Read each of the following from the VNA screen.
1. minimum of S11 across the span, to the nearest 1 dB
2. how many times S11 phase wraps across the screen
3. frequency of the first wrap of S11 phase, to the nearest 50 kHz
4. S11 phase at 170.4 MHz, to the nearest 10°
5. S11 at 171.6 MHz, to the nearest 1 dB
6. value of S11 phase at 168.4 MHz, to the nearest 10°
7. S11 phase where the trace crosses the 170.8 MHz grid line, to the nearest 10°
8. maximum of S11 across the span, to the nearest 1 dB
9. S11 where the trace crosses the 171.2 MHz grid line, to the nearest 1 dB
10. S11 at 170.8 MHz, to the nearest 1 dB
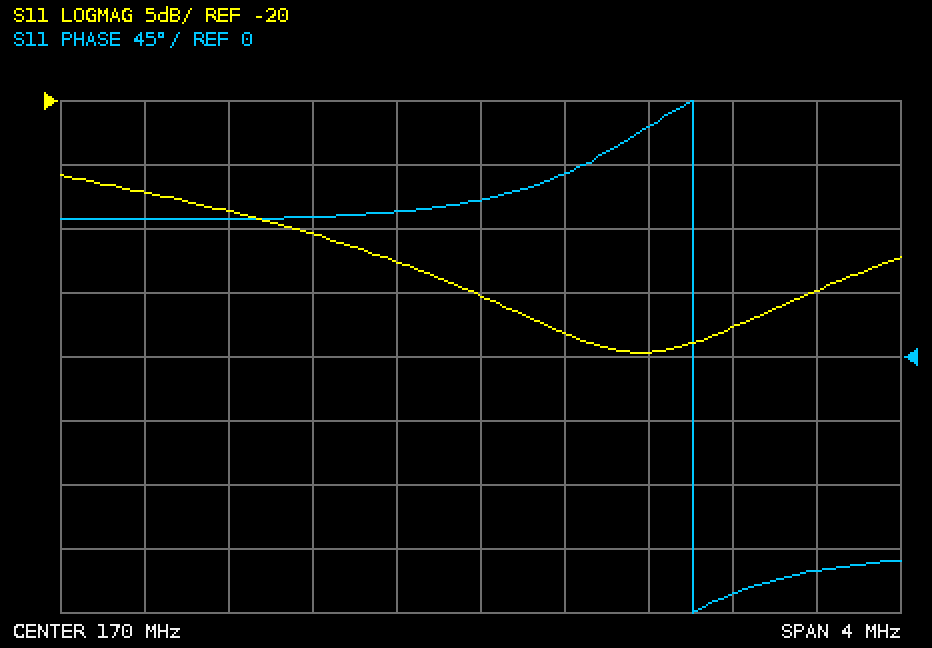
-40 dB
1
171.00 MHz
130°
-35 dB
100°
160°
-26 dB
-38 dB
-40 dB
